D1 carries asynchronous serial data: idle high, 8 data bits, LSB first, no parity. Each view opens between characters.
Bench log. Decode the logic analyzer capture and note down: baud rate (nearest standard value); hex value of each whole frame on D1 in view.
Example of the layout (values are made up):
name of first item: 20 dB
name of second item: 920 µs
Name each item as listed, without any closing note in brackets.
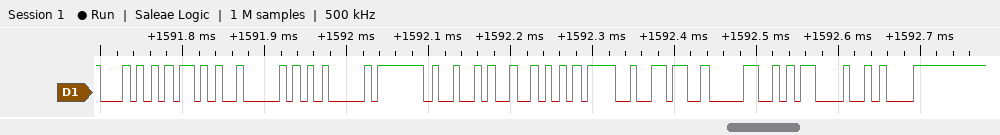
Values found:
baud rate: 115200 baud
hex value of each whole frame on D1 in view: 54, 2B, 50, 41, 49, 52, 3D, 36, 30, 0D, 0A
